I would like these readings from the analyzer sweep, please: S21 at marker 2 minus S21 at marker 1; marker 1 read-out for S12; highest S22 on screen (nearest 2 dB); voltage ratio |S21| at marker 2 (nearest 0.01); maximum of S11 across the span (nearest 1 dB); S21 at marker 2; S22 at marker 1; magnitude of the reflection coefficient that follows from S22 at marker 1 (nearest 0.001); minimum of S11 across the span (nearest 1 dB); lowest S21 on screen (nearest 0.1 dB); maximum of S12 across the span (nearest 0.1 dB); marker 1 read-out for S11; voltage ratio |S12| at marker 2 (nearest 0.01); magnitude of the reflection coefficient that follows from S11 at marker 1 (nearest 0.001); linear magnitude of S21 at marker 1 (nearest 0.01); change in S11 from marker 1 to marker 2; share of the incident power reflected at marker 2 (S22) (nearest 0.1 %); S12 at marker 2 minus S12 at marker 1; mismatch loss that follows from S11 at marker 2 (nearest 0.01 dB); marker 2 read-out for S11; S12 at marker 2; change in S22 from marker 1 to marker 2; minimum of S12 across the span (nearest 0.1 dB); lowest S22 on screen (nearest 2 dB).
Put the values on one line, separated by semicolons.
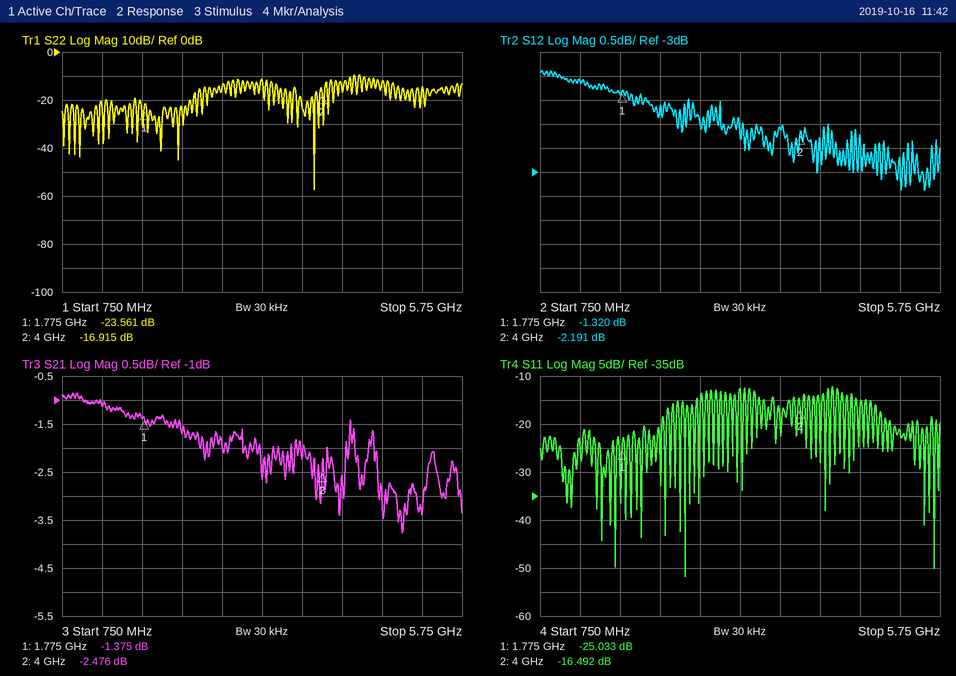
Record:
-1.101 dB; -1.320 dB; -10 dB; 0.75; -12 dB; -2.476 dB; -23.561 dB; 0.066; -52 dB; -3.8 dB; -0.9 dB; -25.033 dB; 0.78; 0.056; 0.85; 8.541 dB; 2.0 %; -0.871 dB; 0.10 dB; -16.492 dB; -2.191 dB; 6.646 dB; -3.4 dB; -58 dB
